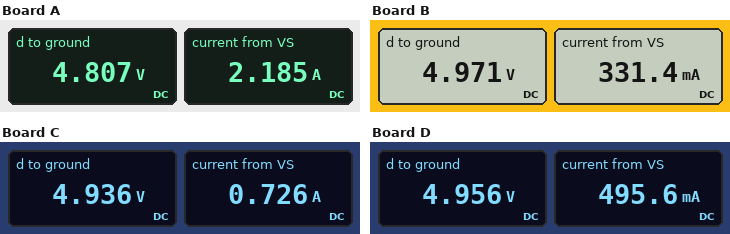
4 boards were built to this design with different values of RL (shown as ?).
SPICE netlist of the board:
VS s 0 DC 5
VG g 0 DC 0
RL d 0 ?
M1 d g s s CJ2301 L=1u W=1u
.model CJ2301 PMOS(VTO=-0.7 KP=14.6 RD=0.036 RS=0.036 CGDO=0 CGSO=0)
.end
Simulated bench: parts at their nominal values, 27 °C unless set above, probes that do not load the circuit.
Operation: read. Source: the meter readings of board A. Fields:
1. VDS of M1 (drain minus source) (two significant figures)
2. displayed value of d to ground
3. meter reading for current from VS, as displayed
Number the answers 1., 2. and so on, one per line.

1. -190 mV
2. 4.807 V
3. 2.185 A
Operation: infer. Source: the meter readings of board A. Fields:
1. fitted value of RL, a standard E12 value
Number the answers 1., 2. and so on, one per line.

1. 2.2 Ω
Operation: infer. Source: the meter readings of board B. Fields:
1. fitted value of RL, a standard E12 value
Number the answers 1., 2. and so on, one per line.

1. 15 Ω
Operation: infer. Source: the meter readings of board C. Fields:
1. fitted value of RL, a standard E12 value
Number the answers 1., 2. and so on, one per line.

1. 6.8 Ω
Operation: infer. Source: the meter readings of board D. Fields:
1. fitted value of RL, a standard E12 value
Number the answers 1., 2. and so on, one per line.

1. 10 Ω
